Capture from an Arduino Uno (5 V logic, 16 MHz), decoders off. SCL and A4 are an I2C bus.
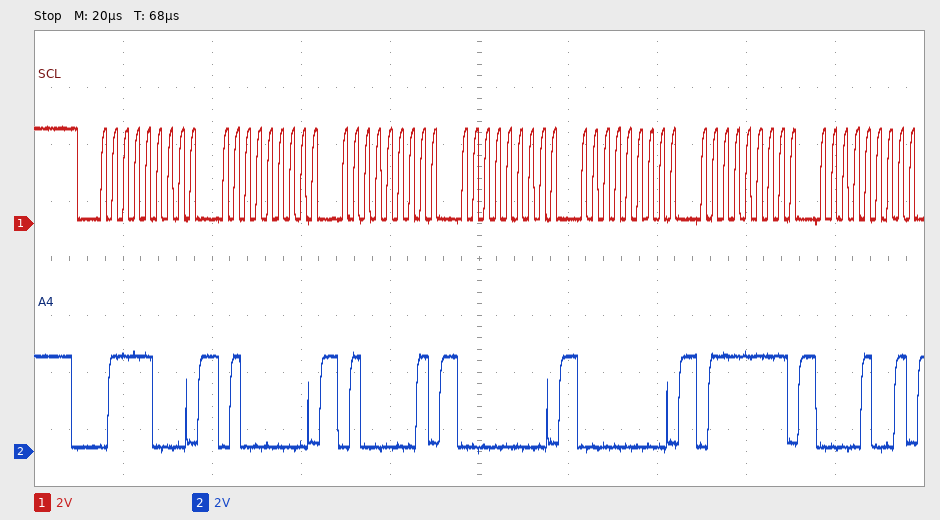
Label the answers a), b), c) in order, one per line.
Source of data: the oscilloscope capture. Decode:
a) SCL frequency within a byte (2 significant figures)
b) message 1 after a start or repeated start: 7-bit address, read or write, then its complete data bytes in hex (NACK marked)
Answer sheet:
a) 400 kHz
b) 0x3C write: 40 41 00 00 7F 09
